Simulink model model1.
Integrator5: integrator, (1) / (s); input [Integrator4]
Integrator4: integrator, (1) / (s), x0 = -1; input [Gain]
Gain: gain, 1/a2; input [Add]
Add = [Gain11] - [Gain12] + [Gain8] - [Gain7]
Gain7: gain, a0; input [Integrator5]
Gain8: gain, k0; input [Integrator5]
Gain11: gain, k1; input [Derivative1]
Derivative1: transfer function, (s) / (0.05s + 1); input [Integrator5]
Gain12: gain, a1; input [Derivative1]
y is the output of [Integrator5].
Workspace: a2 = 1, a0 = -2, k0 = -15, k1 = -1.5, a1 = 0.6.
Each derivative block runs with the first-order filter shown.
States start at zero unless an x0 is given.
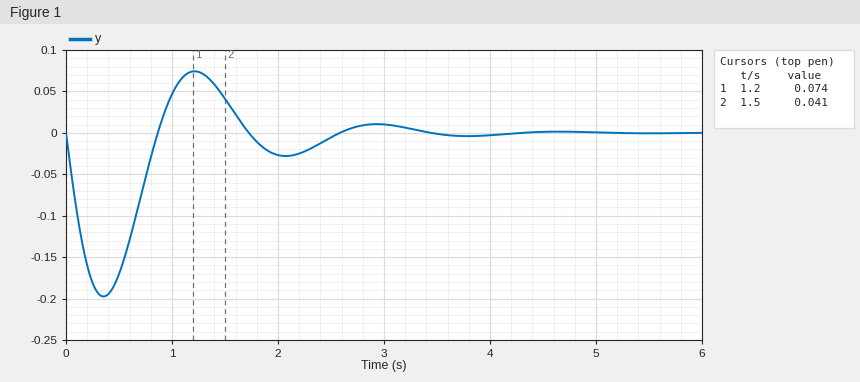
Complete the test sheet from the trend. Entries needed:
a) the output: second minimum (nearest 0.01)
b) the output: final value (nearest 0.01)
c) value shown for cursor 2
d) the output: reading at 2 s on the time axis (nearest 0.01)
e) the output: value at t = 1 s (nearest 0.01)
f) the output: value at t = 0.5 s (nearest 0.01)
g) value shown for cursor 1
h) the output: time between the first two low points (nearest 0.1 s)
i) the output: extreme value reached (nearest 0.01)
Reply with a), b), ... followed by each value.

a) -0.03
b) 0.00
c) 0.041
d) -0.03
e) 0.05
f) -0.17
g) 0.074
h) 1.7 s
i) -0.20
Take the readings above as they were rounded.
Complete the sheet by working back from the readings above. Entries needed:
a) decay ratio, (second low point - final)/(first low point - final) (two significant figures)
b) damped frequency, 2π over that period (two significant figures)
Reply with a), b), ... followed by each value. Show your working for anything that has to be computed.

a) (-0.03 - 0) / (-0.2 - 0) = 0.15
b) 2π / 1.7 = 3.7 rad/s
